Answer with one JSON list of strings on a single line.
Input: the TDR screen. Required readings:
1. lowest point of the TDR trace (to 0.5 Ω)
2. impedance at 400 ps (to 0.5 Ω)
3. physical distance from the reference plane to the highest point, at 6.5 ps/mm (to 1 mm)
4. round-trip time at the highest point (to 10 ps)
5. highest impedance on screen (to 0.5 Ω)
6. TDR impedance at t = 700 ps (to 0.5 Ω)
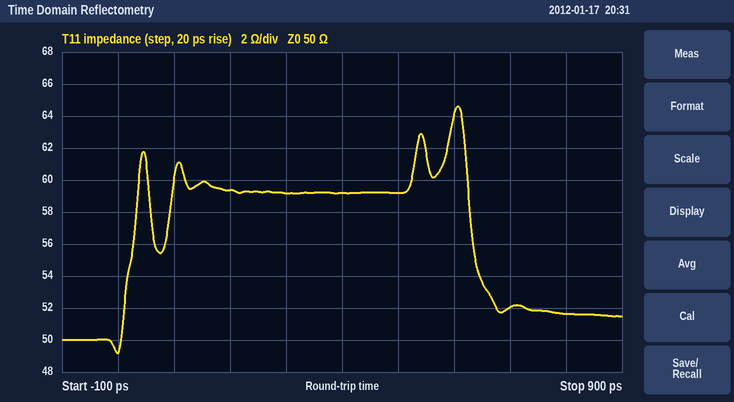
["49.0 Ω", "59.0 Ω", "47 mm", "610 ps", "64.5 Ω", "52.0 Ω"]
